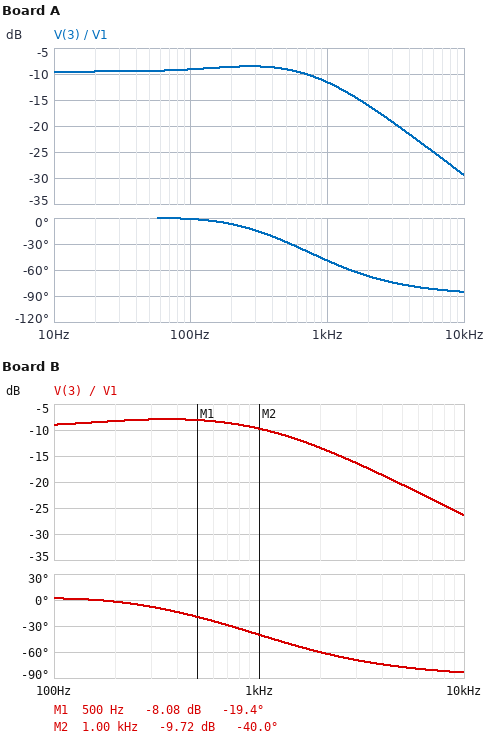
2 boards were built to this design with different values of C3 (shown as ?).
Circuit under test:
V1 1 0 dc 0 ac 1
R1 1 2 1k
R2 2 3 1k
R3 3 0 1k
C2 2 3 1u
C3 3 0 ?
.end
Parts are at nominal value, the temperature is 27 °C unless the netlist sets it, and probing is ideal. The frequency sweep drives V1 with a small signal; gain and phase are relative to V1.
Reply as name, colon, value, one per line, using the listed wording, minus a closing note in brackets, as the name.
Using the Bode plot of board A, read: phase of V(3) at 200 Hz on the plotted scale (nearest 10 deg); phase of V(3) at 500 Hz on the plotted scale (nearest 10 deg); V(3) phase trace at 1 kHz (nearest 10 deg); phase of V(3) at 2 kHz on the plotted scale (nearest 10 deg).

phase of V(3) at 200 Hz on the plotted scale: -10 deg
phase of V(3) at 500 Hz on the plotted scale: -30 deg
V(3) phase trace at 1 kHz: -50 deg
phase of V(3) at 2 kHz on the plotted scale: -70 deg
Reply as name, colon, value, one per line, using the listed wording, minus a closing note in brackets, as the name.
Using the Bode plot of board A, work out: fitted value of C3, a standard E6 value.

fitted value of C3, a standard E6 value: 470 nF
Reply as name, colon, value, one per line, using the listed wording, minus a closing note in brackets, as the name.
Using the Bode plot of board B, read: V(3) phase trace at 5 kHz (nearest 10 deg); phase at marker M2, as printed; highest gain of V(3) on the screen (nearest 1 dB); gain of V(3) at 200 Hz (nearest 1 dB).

V(3) phase trace at 5 kHz: -80 deg
phase at marker M2, as printed: -40.0 deg
highest gain of V(3) on the screen: -8 dB
gain of V(3) at 200 Hz: -8 dB
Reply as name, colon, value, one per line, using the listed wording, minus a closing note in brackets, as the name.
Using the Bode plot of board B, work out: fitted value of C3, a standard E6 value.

fitted value of C3, a standard E6 value: 330 nF
